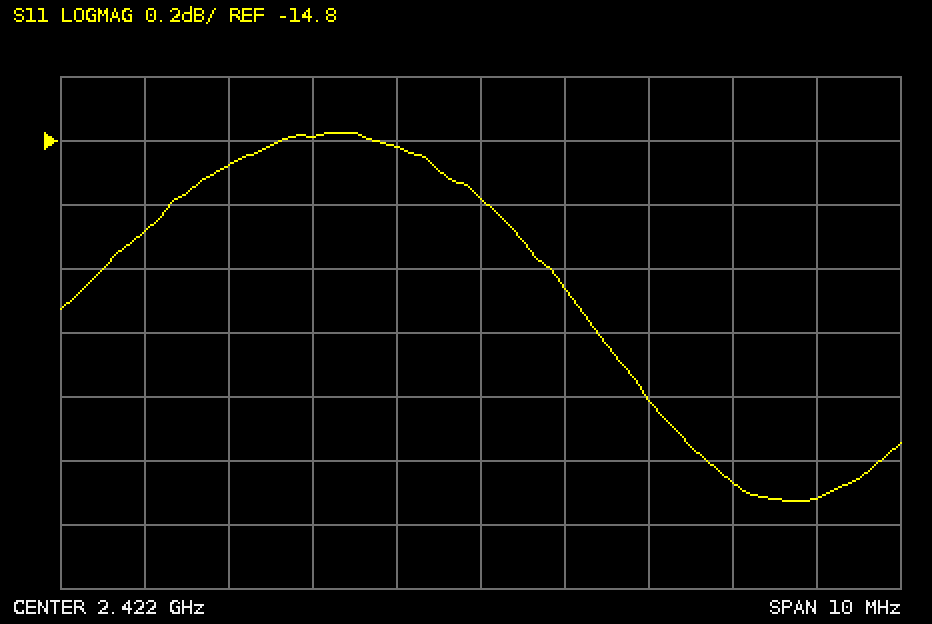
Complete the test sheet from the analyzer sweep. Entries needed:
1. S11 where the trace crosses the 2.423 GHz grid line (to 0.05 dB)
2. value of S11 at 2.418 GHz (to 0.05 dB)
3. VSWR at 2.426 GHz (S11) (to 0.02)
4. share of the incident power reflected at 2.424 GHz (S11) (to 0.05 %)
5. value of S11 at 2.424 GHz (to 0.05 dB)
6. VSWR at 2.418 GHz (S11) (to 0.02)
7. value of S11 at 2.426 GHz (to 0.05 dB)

-15.25 dB
-15.10 dB
1.38
2.75 %
-15.60 dB
1.42
-15.90 dB
